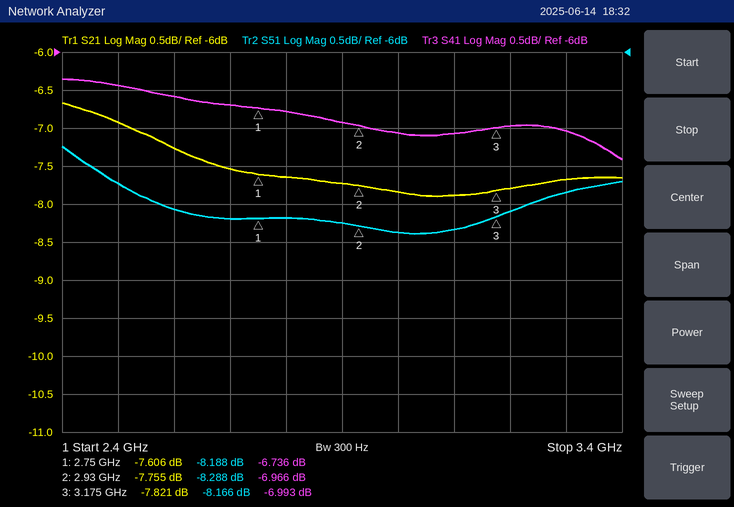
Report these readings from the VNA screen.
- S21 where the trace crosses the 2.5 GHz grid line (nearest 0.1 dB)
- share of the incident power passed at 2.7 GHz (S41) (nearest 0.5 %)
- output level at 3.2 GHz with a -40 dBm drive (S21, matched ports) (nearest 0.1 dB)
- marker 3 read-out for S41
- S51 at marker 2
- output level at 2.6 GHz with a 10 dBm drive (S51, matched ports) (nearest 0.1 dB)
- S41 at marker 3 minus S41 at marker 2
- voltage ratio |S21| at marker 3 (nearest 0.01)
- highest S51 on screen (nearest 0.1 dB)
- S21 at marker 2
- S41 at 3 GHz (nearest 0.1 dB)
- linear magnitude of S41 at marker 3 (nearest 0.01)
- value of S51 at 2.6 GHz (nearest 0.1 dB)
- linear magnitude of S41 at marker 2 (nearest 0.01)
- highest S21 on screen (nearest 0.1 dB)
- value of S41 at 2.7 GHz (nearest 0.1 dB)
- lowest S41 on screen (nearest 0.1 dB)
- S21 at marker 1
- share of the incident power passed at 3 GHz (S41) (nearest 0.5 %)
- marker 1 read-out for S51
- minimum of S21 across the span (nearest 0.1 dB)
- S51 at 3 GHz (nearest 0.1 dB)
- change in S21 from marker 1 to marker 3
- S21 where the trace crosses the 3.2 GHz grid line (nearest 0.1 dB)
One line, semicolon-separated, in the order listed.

-6.9 dB; 21.5 %; -47.8 dBm; -6.993 dB; -8.288 dB; 1.9 dBm; -0.027 dB; 0.41; -7.2 dB; -7.755 dB; -7.1 dB; 0.45; -8.1 dB; 0.45; -6.7 dB; -6.7 dB; -7.4 dB; -7.606 dB; 19.5 %; -8.188 dB; -7.9 dB; -8.4 dB; -0.215 dB; -7.8 dB
